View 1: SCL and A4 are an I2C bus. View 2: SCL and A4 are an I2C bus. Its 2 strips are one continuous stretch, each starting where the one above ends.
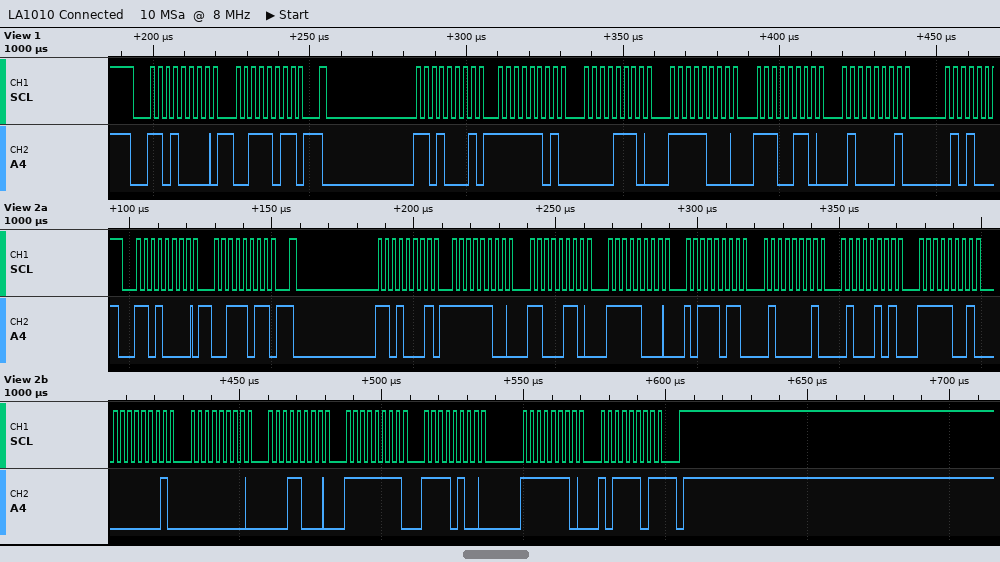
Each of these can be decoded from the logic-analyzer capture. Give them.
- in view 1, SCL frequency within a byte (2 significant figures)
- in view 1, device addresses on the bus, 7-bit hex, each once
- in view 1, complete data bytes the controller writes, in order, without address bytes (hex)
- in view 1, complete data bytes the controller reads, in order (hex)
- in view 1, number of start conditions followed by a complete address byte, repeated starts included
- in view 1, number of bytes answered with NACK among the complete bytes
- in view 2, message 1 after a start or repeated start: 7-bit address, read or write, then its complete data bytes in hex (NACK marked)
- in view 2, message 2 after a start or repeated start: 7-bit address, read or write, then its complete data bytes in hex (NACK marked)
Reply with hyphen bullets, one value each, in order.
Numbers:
- 400 kHz
- 0x68
- 3B
- FD 0E F8 E6 41
- 2
- 0
- 0x68 write: 3B
- 0x68 read: FC C6 F8 BB 41 45 F9 01 00 18 FF F4 FE BD NACK
